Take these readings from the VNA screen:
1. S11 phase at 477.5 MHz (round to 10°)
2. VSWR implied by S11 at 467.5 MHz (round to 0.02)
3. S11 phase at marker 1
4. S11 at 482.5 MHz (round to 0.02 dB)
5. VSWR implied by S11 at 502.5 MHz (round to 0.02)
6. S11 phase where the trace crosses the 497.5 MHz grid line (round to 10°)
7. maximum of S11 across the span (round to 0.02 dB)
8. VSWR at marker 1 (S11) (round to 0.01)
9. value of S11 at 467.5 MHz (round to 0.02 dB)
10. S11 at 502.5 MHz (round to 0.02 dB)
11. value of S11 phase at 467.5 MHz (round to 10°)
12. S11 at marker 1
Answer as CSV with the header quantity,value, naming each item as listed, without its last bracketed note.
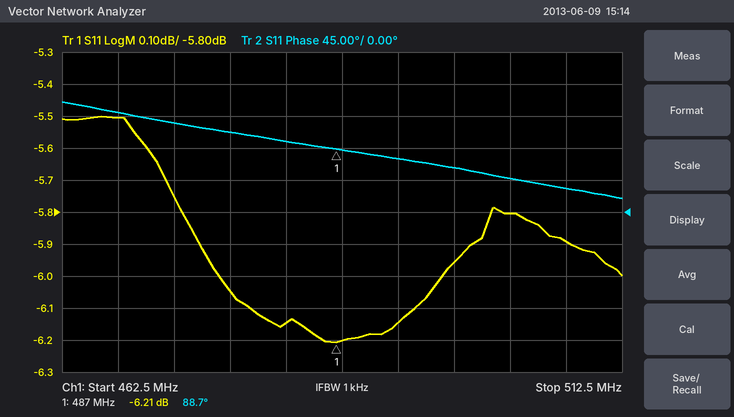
quantity,value
S11 phase at 477.5 MHz,110°
VSWR implied by S11 at 467.5 MHz,3.26
S11 phase at marker 1,88.7°
S11 at 482.5 MHz,-6.14 dB
VSWR implied by S11 at 502.5 MHz,3.10
S11 phase where the trace crosses the 497.5 MHz grid line,60°
maximum of S11 across the span,-5.50 dB
VSWR at marker 1 (S11),2.92
value of S11 at 467.5 MHz,-5.50 dB
S11 at 502.5 MHz,-5.80 dB
value of S11 phase at 467.5 MHz,140°
S11 at marker 1,-6.21 dB
